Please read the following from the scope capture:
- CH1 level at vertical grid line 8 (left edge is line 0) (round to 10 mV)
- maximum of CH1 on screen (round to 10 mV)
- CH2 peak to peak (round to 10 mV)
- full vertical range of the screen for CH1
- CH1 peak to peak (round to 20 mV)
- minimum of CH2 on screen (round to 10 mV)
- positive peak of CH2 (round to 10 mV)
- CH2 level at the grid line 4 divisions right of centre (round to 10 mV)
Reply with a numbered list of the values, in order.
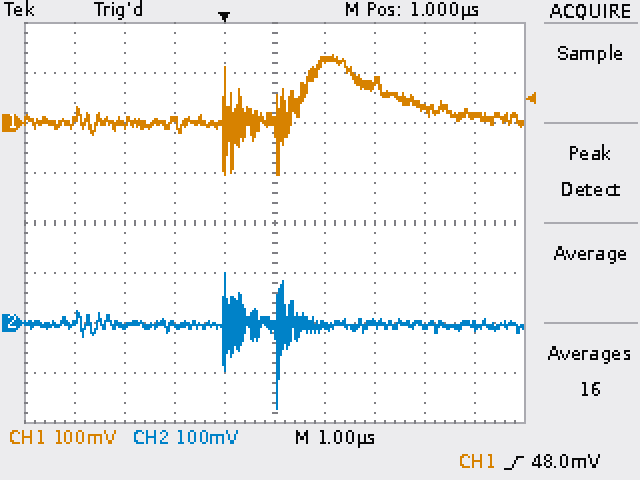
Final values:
1. 30 mV
2. 140 mV
3. 270 mV
4. 800 mV
5. 240 mV
6. -170 mV
7. 100 mV
8. -10 mV
